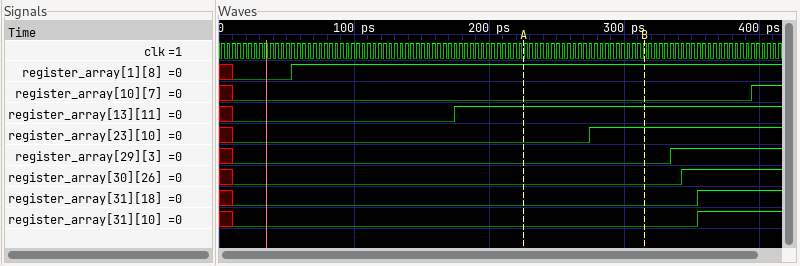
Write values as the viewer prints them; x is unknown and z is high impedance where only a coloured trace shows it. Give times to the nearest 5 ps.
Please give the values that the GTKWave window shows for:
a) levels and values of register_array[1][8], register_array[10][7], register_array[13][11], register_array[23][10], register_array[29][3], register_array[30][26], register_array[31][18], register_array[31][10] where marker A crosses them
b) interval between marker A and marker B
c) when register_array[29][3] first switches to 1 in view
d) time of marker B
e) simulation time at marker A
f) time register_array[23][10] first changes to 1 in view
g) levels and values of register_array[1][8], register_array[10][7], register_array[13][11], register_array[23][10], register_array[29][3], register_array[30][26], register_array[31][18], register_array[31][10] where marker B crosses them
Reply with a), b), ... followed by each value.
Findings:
a) register_array[1][8]=1, register_array[10][7]=0, register_array[13][11]=1, register_array[23][10]=0, register_array[29][3]=0, register_array[30][26]=0, register_array[31][18]=0, register_array[31][10]=0
b) 90 ps
c) 335 ps
d) 315 ps
e) 225 ps
f) 275 ps
g) register_array[1][8]=1, register_array[10][7]=0, register_array[13][11]=1, register_array[23][10]=1, register_array[29][3]=0, register_array[30][26]=0, register_array[31][18]=0, register_array[31][10]=0
